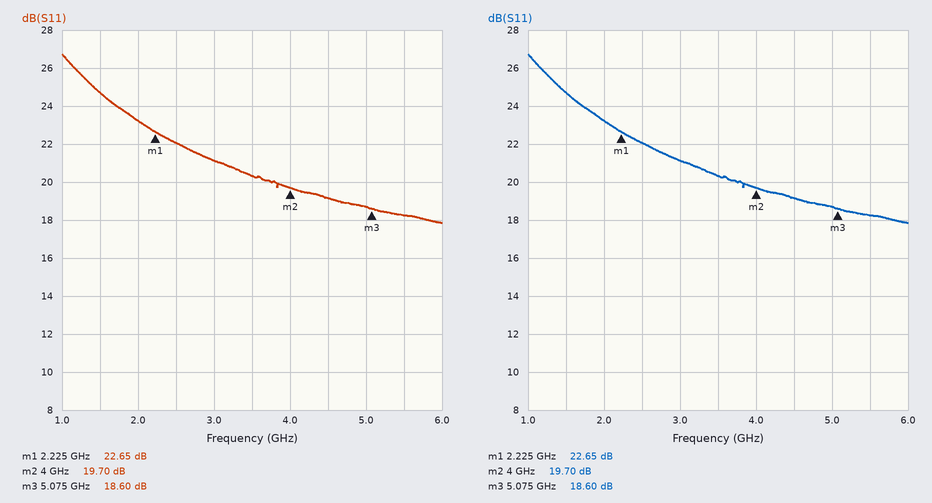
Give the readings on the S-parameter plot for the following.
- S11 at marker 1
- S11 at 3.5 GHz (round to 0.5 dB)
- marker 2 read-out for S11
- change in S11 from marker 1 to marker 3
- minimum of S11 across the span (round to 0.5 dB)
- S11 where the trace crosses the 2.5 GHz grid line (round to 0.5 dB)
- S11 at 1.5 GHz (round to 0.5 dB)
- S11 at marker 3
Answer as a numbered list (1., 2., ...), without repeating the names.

1. 22.65 dB
2. 20.5 dB
3. 19.70 dB
4. -4.05 dB
5. 18.0 dB
6. 22.0 dB
7. 24.5 dB
8. 18.60 dB
